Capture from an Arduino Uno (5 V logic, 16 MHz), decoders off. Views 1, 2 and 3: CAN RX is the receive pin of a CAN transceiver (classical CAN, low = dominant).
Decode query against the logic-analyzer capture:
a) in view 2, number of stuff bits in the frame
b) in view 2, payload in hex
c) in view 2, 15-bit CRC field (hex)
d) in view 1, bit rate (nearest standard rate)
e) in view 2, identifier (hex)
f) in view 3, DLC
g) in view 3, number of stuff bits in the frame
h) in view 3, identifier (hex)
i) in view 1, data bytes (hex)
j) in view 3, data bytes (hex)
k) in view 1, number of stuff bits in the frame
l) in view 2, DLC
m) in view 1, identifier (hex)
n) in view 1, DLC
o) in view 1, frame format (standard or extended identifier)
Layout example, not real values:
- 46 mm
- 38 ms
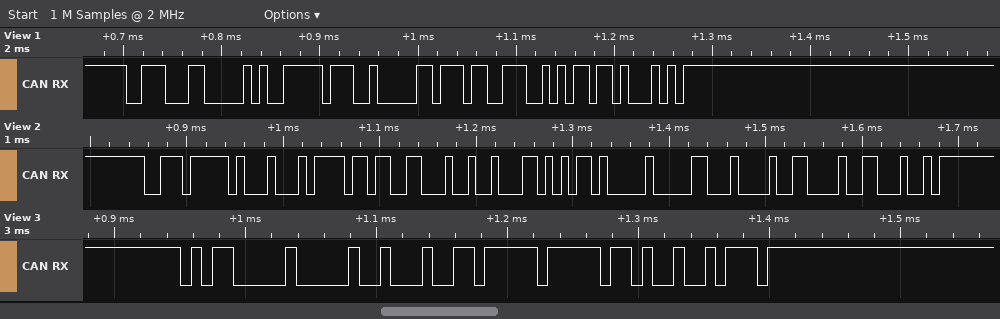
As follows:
- 3
- BD B3 12 46 AD 00 22 13
- 0x04C4
- 125 kbit/s
- 0x3BF
- 2
- 4
- 0x580
- FF 20 BB 39
- 26 FF
- 3
- 8
- 0x38C
- 4
- standard
